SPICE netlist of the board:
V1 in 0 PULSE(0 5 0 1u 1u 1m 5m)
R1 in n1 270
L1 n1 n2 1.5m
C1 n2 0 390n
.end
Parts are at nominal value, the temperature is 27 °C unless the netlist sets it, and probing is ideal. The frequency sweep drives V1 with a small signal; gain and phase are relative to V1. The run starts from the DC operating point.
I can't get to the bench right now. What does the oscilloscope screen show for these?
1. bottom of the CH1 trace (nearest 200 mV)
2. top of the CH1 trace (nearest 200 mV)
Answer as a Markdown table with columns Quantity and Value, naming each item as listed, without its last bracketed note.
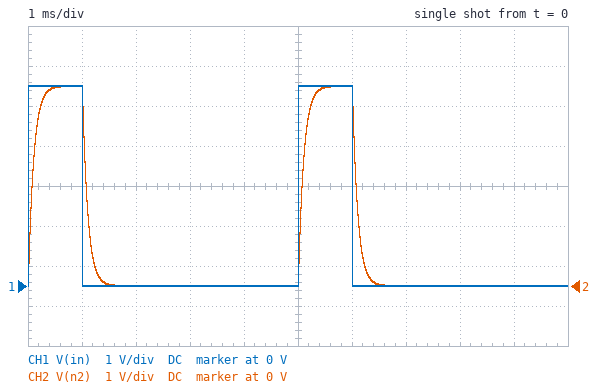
| Quantity | Value |
|---|---|
| bottom of the CH1 trace | 0 V |
| top of the CH1 trace | 5.0 V |
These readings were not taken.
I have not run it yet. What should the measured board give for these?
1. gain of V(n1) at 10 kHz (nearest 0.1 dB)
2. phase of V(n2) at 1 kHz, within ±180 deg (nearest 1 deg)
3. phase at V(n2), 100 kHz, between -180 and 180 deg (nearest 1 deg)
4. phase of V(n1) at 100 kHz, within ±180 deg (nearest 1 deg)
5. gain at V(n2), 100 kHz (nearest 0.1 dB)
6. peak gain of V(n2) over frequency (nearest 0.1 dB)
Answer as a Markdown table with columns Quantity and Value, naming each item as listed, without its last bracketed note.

| Quantity | Value |
|---|---|
| gain of V(n1) at 10 kHz | -14.2 dB |
| phase of V(n2) at 1 kHz, within ±180 deg | -34 deg |
| phase at V(n2), 100 kHz, between -180 and 180 deg | -164 deg |
| phase of V(n1) at 100 kHz, within ±180 deg | 16 deg |
| gain at V(n2), 100 kHz | -47.6 dB |
| peak gain of V(n2) over frequency | 0 dB |
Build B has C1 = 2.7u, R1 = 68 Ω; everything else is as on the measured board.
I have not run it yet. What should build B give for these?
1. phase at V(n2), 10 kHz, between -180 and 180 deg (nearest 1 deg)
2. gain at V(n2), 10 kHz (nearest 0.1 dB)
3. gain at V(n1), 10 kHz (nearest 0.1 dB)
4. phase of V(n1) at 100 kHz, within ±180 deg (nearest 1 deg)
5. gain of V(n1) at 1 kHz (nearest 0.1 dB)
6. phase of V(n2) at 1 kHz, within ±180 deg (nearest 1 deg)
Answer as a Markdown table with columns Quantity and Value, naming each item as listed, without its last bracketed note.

| Quantity | Value |
|---|---|
| phase at V(n2), 10 kHz, between -180 and 180 deg | -142 deg |
| gain at V(n2), 10 kHz | -25.5 dB |
| gain at V(n1), 10 kHz | -2.0 dB |
| phase of V(n1) at 100 kHz, within ±180 deg | 4 deg |
| gain of V(n1) at 1 kHz | -4.6 dB |
| phase of V(n2) at 1 kHz, within ±180 deg | -54 deg |
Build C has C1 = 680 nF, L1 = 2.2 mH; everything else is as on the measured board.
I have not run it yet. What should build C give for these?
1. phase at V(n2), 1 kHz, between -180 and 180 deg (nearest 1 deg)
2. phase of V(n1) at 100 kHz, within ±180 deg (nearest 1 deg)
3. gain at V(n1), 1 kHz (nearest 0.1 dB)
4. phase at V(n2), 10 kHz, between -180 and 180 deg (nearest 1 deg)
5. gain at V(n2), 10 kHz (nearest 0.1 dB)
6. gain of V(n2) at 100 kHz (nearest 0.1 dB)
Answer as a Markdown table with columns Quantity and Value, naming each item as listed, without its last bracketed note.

| Quantity | Value |
|---|---|
| phase at V(n2), 1 kHz, between -180 and 180 deg | -51 deg |
| phase of V(n1) at 100 kHz, within ±180 deg | 11 deg |
| gain at V(n1), 1 kHz | -4.0 dB |
| phase at V(n2), 10 kHz, between -180 and 180 deg | -113 deg |
| gain at V(n2), 10 kHz | -22.0 dB |
| gain of V(n2) at 100 kHz | -55.6 dB |
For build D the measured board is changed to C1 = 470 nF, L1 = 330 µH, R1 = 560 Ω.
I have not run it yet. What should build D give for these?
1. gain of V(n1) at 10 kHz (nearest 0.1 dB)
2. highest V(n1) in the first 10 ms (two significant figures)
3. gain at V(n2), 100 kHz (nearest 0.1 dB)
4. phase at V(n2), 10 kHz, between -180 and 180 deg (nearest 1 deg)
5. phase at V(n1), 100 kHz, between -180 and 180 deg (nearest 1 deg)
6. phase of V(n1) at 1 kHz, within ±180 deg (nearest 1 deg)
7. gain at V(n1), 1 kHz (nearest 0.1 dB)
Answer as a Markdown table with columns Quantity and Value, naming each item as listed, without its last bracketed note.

| Quantity | Value |
|---|---|
| gain of V(n1) at 10 kHz | -32.6 dB |
| highest V(n1) in the first 10 ms | 4.9 V |
| gain at V(n2), 100 kHz | -44.9 dB |
| phase at V(n2), 10 kHz, between -180 and 180 deg | -89 deg |
| phase at V(n1), 100 kHz, between -180 and 180 deg | 70 deg |
| phase of V(n1) at 1 kHz, within ±180 deg | -59 deg |
| gain at V(n1), 1 kHz | -5.8 dB |
